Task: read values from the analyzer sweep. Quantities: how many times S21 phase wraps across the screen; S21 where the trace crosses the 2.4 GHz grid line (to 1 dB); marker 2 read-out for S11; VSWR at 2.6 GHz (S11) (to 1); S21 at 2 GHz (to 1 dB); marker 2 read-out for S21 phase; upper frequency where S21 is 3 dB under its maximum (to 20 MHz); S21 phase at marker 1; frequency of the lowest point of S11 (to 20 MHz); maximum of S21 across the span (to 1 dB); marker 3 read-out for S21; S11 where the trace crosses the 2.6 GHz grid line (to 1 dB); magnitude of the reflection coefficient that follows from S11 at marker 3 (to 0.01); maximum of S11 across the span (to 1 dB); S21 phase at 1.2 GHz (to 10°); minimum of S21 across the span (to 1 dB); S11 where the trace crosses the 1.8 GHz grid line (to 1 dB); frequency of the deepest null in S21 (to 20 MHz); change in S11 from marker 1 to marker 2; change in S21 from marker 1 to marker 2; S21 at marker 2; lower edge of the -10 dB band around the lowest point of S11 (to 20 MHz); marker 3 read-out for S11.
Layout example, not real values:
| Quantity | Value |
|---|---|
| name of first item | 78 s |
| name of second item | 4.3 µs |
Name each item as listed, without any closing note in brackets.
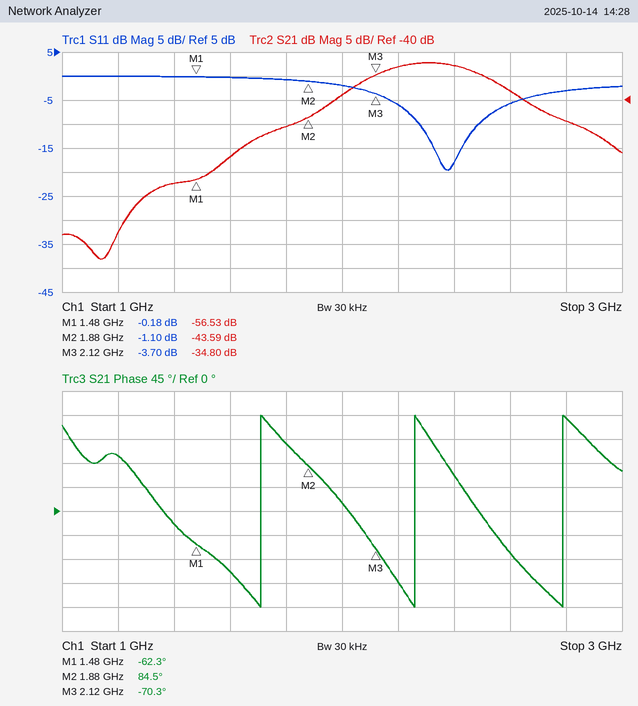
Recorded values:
| Quantity | Value |
|---|---|
| how many times S21 phase wraps across the screen | 3 |
| S21 where the trace crosses the 2.4 GHz grid line | -33 dB |
| marker 2 read-out for S11 | -1.10 dB |
| VSWR at 2.6 GHz (S11) | 3 |
| S21 at 2 GHz | -39 dB |
| marker 2 read-out for S21 phase | 84.5° |
| upper frequency where S21 is 3 dB under its maximum | 2.52 GHz |
| S21 phase at marker 1 | -62.3° |
| frequency of the lowest point of S11 | 2.38 GHz |
| maximum of S21 across the span | -32 dB |
| marker 3 read-out for S21 | -34.80 dB |
| S11 where the trace crosses the 2.6 GHz grid line | -6 dB |
| magnitude of the reflection coefficient that follows from S11 at marker 3 | 0.65 |
| maximum of S11 across the span | 0 dB |
| S21 phase at 1.2 GHz | 100° |
| minimum of S21 across the span | -73 dB |
| S11 where the trace crosses the 1.8 GHz grid line | -1 dB |
| frequency of the deepest null in S21 | 1.14 GHz |
| change in S11 from marker 1 to marker 2 | -0.92 dB |
| change in S21 from marker 1 to marker 2 | 12.94 dB |
| S21 at marker 2 | -43.59 dB |
| lower edge of the -10 dB band around the lowest point of S11 | 2.28 GHz |
| marker 3 read-out for S11 | -3.70 dB |
